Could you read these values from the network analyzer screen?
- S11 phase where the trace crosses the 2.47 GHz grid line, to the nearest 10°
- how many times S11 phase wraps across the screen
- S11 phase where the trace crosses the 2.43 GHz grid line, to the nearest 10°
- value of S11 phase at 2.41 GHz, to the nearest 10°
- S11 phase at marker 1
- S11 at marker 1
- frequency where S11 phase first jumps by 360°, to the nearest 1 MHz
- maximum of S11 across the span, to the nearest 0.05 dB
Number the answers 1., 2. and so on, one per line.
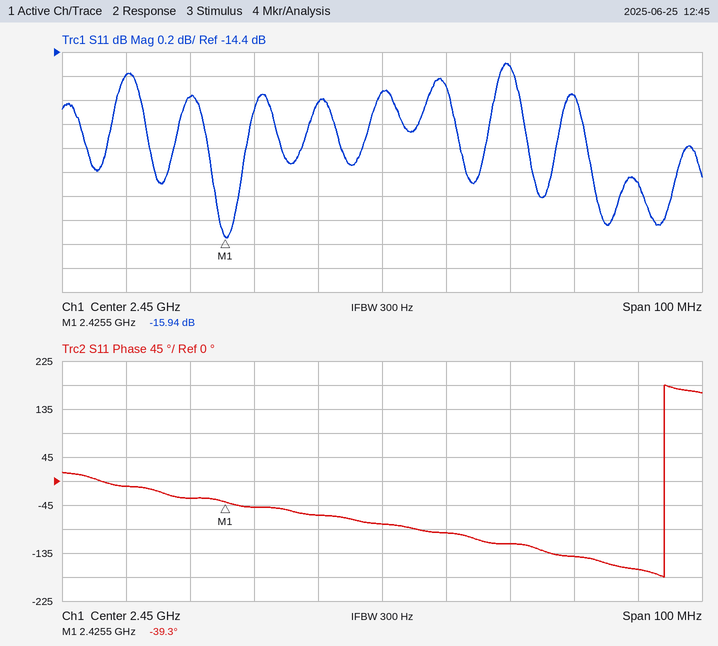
1. -120°
2. 1
3. -50°
4. -10°
5. -39.3°
6. -15.94 dB
7. 2.494 GHz
8. -14.50 dB
